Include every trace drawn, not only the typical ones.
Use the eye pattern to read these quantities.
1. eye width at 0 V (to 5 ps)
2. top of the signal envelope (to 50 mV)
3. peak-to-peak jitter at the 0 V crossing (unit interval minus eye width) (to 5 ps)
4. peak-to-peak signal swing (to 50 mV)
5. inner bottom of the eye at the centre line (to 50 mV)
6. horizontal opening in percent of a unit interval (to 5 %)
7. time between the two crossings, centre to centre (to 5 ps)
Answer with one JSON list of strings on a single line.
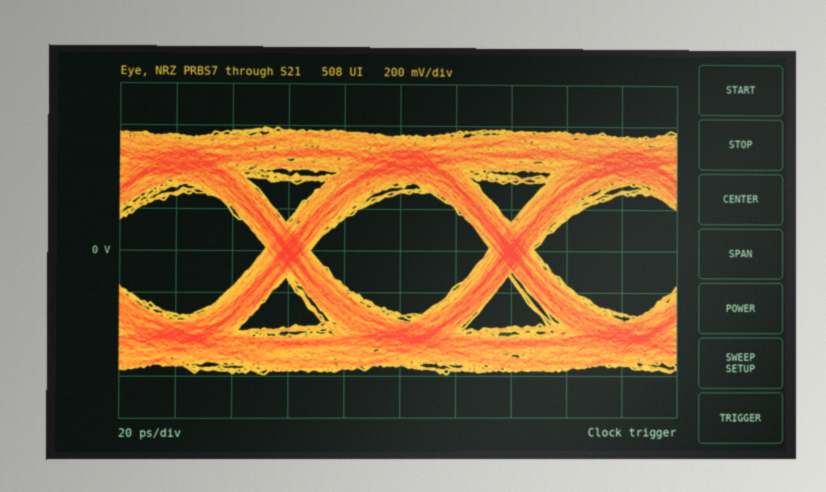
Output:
["65 ps", "600 mV", "15 ps", "1.20 V", "-300 mV", "80 %", "80 ps"]
